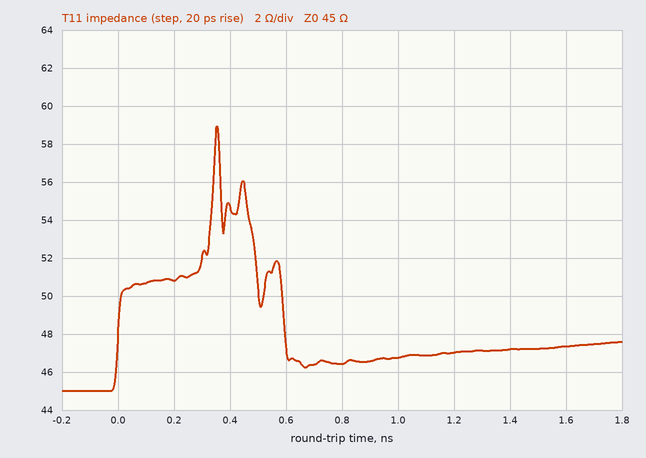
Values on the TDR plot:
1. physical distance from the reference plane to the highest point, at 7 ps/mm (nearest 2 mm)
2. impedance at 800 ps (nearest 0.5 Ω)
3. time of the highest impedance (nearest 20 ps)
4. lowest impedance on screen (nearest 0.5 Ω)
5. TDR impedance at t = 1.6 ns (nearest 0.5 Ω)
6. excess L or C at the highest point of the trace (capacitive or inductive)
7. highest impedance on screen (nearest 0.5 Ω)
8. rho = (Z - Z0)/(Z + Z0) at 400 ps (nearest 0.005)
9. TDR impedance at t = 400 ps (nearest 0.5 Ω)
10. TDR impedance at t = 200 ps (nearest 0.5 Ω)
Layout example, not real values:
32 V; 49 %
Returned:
26 mm; 46.5 Ω; 360 ps; 45.0 Ω; 47.5 Ω; inductive; 59.0 Ω; +0.095; 54.5 Ω; 51.0 Ω
